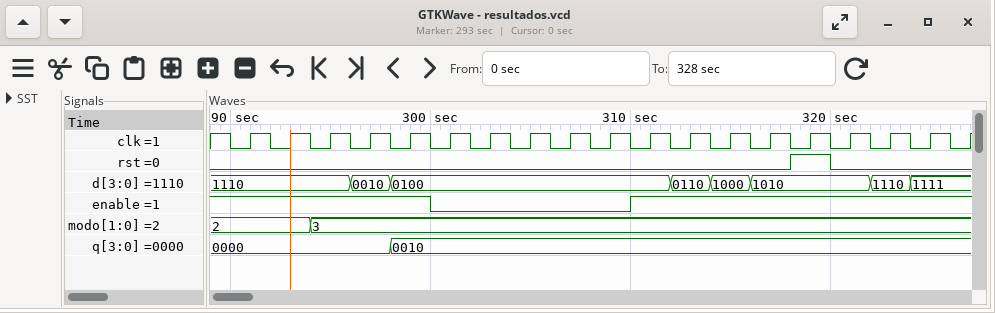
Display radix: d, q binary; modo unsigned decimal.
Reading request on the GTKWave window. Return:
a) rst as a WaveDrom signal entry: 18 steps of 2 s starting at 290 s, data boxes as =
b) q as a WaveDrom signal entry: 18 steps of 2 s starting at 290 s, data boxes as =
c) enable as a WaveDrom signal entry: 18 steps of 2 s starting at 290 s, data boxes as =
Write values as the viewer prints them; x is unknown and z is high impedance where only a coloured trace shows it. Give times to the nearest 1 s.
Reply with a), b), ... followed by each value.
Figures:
a) {name: 'rst', wave: '0.............10..'}
b) {name: 'q', wave: '=...=.............', data: '0000 0010'}
c) {name: 'enable', wave: '1....0....1.......'}
